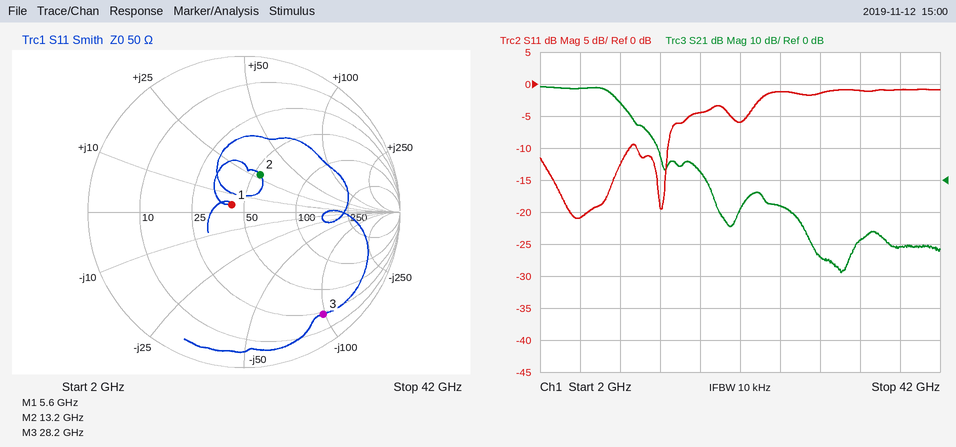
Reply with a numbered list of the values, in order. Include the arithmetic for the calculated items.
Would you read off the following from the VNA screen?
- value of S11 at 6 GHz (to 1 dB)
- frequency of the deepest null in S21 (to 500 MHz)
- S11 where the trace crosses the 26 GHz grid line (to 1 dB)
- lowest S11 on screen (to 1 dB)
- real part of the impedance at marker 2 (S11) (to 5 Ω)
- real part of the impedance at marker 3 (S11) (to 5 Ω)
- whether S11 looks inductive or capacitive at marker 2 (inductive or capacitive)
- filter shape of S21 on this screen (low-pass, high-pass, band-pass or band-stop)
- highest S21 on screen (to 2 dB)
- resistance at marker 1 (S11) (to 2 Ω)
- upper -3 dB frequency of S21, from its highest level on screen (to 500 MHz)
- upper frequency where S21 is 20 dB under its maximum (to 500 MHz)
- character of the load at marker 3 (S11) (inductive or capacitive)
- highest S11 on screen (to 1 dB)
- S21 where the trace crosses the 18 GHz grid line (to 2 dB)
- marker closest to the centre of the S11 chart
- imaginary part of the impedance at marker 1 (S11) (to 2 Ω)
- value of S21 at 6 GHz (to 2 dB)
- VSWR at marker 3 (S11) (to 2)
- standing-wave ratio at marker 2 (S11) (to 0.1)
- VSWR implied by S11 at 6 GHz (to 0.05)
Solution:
1. -21 dB
2. 32.0 GHz
3. -1 dB
4. -21 dB
5. 55 Ω
6. 25 Ω
7. inductive
8. low-pass
9. 30 dB
10. 42 Ω
11. 9.5 GHz
12. 14.0 GHz
13. capacitive
14. -1 dB
15. 2 dB
16. marker 1
17. +4 Ω
18. 28 dB
19. 10
20. 1.7
21. |Γ| = 10^(-21/20) = 0.0891; VSWR = (1 + 0.0891)/(1 − 0.0891) ≈ 1.20
